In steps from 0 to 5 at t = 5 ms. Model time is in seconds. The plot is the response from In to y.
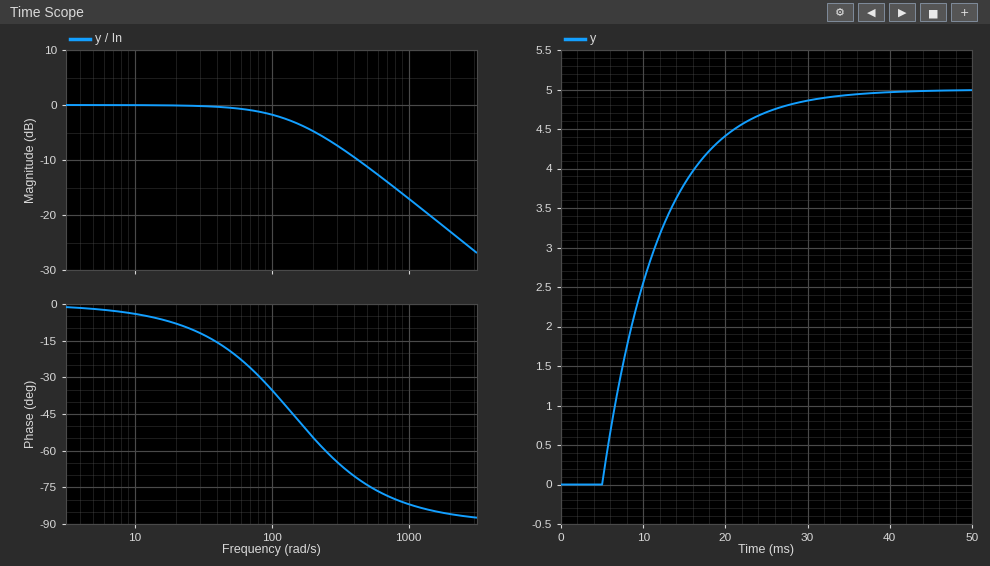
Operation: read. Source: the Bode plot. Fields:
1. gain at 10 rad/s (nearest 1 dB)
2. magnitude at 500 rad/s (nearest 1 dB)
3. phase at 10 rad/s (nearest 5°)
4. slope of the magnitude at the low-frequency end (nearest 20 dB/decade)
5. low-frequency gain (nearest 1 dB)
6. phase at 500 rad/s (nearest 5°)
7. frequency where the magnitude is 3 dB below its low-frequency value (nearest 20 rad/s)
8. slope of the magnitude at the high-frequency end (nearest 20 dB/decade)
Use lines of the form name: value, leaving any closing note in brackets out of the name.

gain at 10 rad/s: 0 dB
magnitude at 500 rad/s: -11 dB
phase at 10 rad/s: -5°
slope of the magnitude at the low-frequency end: 0 dB/decade
low-frequency gain: 0 dB
phase at 500 rad/s: -75°
frequency where the magnitude is 3 dB below its low-frequency value: 140 rad/s
slope of the magnitude at the high-frequency end: -20 dB/decade
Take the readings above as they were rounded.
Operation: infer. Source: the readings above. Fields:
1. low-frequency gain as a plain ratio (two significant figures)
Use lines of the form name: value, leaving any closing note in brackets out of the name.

low-frequency gain as a plain ratio: 1.0
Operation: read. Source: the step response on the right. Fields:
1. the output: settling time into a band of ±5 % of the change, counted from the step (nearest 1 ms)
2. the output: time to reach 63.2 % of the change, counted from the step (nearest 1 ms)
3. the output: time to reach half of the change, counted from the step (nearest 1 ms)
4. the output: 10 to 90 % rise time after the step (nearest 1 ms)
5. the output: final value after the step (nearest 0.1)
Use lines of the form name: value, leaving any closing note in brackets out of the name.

the output: settling time into a band of ±5 % of the change, counted from the step: 21 ms
the output: time to reach 63.2 % of the change, counted from the step: 7 ms
the output: time to reach half of the change, counted from the step: 5 ms
the output: 10 to 90 % rise time after the step: 15 ms
the output: final value after the step: 5.0
